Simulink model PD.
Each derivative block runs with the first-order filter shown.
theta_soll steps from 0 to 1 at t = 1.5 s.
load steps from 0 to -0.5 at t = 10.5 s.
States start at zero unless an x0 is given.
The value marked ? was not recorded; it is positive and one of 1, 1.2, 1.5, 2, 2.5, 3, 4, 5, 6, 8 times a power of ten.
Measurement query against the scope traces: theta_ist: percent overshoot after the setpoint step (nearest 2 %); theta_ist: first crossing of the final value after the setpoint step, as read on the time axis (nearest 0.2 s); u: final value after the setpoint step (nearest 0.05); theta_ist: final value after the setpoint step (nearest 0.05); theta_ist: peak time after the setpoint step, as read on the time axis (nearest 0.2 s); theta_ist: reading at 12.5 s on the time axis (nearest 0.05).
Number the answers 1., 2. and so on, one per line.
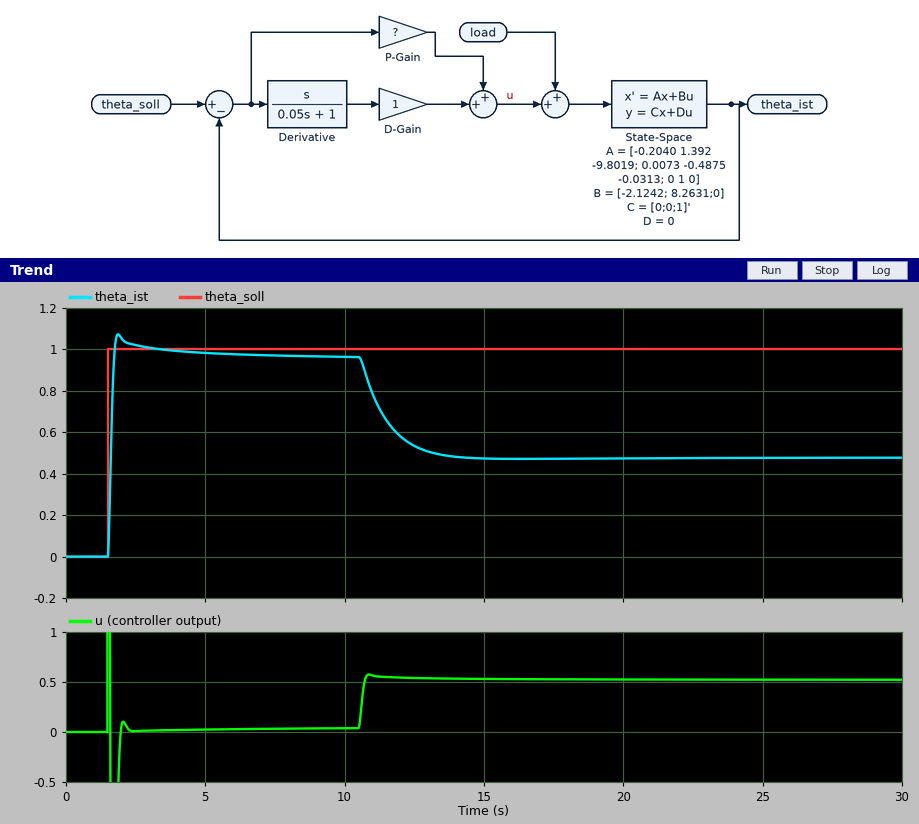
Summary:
1. 12 %
2. 1.8 s
3. 0.05
4. 0.95
5. 1.8 s
6. 0.55
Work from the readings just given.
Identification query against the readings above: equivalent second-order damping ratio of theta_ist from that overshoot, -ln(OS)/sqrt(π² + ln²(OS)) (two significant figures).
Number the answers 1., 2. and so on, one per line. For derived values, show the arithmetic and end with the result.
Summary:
1. ln(0.12) = -2.120; 2.120 / sqrt(9.870 + 4.496) = 0.56
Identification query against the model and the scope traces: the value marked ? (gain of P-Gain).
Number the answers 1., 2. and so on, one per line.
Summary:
1. 1
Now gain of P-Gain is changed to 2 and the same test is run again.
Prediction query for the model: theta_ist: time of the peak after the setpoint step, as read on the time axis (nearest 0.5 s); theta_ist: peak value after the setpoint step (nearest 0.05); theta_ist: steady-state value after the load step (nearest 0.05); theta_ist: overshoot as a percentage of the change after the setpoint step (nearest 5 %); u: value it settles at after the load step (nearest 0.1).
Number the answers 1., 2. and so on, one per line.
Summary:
1. 2.0 s
2. 1.15
3. 0.75
4. 20 %
5. 0.5
